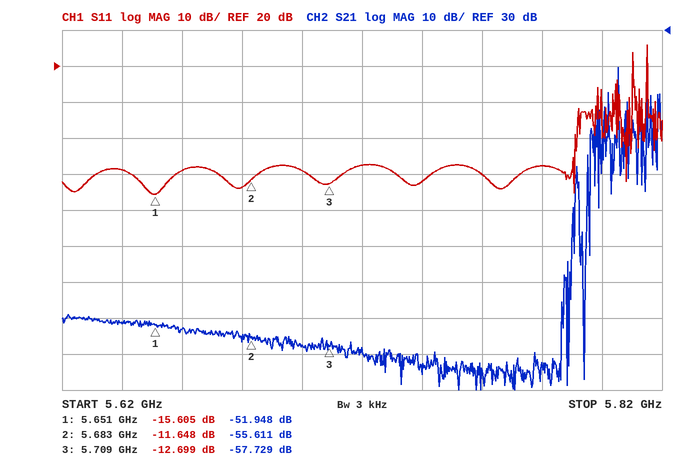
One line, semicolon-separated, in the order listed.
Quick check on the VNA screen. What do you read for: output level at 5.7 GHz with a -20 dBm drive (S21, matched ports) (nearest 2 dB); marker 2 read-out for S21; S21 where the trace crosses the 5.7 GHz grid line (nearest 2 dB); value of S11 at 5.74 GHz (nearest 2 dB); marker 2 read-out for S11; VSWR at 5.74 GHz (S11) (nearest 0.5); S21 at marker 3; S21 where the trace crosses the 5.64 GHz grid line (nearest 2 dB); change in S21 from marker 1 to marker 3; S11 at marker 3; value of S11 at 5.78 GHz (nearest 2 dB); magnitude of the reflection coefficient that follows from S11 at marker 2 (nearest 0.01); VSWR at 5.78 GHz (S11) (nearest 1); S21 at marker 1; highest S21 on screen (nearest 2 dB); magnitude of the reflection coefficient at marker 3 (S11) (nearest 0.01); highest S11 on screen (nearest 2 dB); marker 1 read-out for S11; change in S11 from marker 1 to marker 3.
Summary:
-78 dBm; -55.611 dB; -58 dB; -12 dB; -11.648 dB; 1.5; -57.729 dB; -52 dB; -5.781 dB; -12.699 dB; -8 dB; 0.26; 2; -51.948 dB; 20 dB; 0.23; 26 dB; -15.605 dB; 2.906 dB
